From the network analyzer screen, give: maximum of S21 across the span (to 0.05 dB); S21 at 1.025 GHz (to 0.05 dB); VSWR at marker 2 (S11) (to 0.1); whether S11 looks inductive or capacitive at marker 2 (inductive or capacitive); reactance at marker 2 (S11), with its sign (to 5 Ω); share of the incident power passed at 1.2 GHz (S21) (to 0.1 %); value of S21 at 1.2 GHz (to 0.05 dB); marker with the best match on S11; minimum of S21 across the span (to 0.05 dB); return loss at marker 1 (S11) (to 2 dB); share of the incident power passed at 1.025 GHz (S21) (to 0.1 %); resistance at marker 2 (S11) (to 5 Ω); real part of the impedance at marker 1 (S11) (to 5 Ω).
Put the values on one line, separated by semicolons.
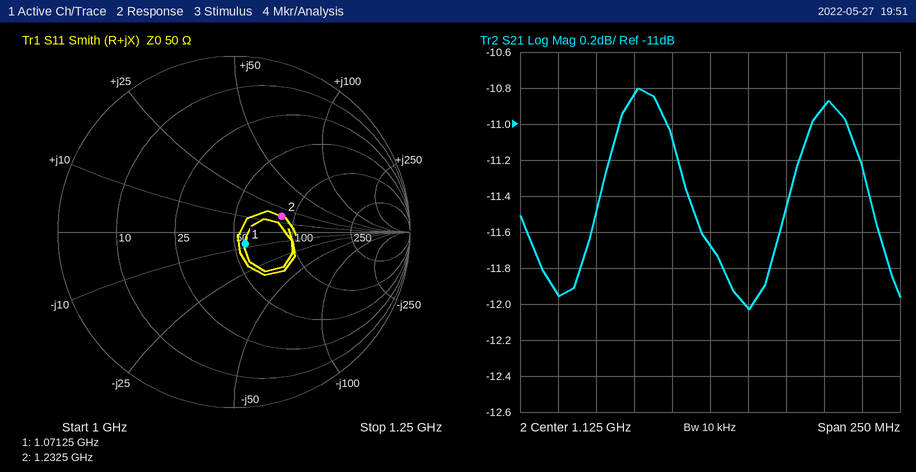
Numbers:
-10.80 dB; -11.95 dB; 1.8; inductive; +15 Ω; 8.1 %; -10.90 dB; marker 1; -12.05 dB; 20 dB; 6.4 %; 85 Ω; 55 Ω
